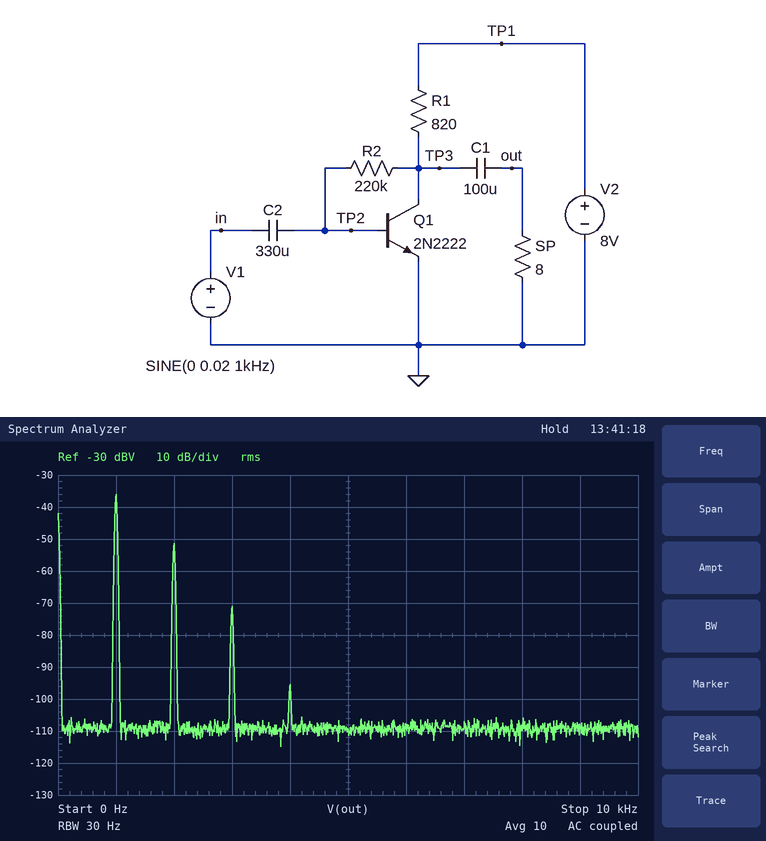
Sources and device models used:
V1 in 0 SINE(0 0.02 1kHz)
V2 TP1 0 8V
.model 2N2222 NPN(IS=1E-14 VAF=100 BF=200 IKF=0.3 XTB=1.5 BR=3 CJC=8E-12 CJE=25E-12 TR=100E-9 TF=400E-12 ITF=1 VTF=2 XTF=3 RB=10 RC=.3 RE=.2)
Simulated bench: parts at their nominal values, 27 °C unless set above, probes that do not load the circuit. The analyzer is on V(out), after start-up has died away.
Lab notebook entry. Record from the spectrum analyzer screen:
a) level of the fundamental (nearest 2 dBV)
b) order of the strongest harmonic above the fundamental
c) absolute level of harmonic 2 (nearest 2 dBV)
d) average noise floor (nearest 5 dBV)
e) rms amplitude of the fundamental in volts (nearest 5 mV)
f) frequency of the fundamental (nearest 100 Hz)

-36 dBV
2
-52 dBV
-110 dBV
15 mV
1.0 kHz
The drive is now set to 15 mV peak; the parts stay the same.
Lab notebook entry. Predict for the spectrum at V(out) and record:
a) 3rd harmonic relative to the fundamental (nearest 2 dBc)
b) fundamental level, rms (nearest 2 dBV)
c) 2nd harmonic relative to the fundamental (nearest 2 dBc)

-40 dBc
-38 dBV
-18 dBc
